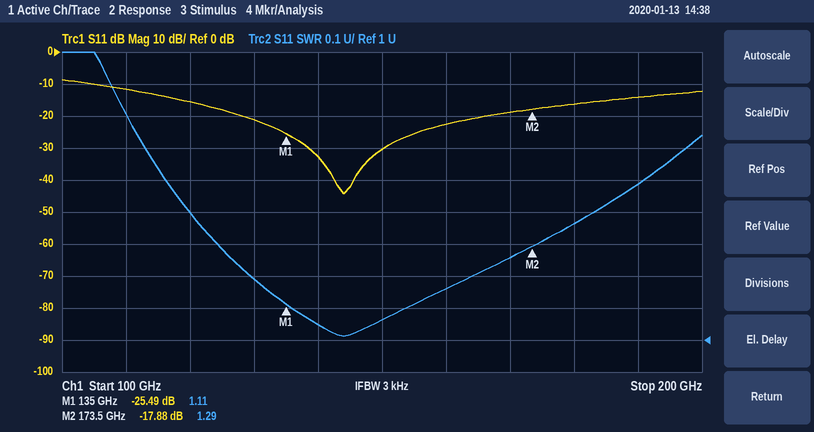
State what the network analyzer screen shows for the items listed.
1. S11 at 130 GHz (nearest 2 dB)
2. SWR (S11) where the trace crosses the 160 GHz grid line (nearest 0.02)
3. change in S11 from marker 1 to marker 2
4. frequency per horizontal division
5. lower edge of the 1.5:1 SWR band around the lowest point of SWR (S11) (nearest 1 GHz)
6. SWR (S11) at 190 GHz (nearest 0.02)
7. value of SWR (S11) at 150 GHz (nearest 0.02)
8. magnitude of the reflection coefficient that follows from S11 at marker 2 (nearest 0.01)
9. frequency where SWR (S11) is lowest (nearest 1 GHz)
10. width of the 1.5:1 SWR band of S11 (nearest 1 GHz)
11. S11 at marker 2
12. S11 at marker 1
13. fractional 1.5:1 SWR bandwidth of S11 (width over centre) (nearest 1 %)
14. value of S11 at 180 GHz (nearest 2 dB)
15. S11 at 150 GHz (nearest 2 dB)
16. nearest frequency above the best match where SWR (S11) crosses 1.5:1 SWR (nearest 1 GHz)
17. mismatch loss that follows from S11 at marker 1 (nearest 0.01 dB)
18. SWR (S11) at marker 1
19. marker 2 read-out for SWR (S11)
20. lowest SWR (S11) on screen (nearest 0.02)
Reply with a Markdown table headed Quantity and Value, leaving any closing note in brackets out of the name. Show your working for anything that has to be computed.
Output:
| Quantity | Value |
|---|---|
| S11 at 130 GHz | -22 dB |
| SWR (S11) where the trace crosses the 160 GHz grid line | 1.16 |
| change in S11 from marker 1 to marker 2 | -17.88 − (-25.49) = 7.61 dB |
| frequency per horizontal division | 10 GHz |
| lower edge of the 1.5:1 SWR band around the lowest point of SWR (S11) | 116 GHz |
| SWR (S11) at 190 GHz | 1.48 |
| value of SWR (S11) at 150 GHz | 1.06 |
| magnitude of the reflection coefficient that follows from S11 at marker 2 | 10^(-17.88/20) ≈ 0.13 |
| frequency where SWR (S11) is lowest | 144 GHz |
| width of the 1.5:1 SWR band of S11 | 191 GHz − 116 GHz = 75 GHz |
| S11 at marker 2 | -17.88 dB |
| S11 at marker 1 | -25.49 dB |
| fractional 1.5:1 SWR bandwidth of S11 (width over centre) | 75 GHz / 153.5 GHz ≈ 49 % |
| value of S11 at 180 GHz | -16 dB |
| S11 at 150 GHz | -30 dB |
| nearest frequency above the best match where SWR (S11) crosses 1.5:1 SWR | 191 GHz |
| mismatch loss that follows from S11 at marker 1 | −10 log10(1 − 10^(-25.49/10)) ≈ 0.01 dB |
| SWR (S11) at marker 1 | 1.11 |
| marker 2 read-out for SWR | 1.29 |
| lowest SWR (S11) on screen | 1.02 |
